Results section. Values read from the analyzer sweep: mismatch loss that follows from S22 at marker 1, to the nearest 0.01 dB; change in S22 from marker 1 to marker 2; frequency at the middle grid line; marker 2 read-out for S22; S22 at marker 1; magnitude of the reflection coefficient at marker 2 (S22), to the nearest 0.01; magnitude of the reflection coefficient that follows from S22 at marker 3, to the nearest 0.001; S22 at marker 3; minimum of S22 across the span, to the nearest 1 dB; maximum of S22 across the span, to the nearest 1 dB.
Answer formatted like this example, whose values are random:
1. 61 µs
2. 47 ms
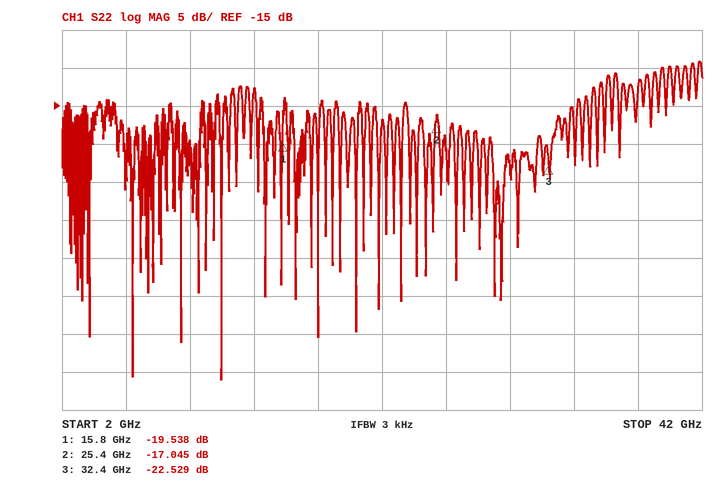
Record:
1. 0.05 dB
2. 2.493 dB
3. 22 GHz
4. -17.045 dB
5. -19.538 dB
6. 0.14
7. 0.075
8. -22.529 dB
9. -51 dB
10. -9 dB
